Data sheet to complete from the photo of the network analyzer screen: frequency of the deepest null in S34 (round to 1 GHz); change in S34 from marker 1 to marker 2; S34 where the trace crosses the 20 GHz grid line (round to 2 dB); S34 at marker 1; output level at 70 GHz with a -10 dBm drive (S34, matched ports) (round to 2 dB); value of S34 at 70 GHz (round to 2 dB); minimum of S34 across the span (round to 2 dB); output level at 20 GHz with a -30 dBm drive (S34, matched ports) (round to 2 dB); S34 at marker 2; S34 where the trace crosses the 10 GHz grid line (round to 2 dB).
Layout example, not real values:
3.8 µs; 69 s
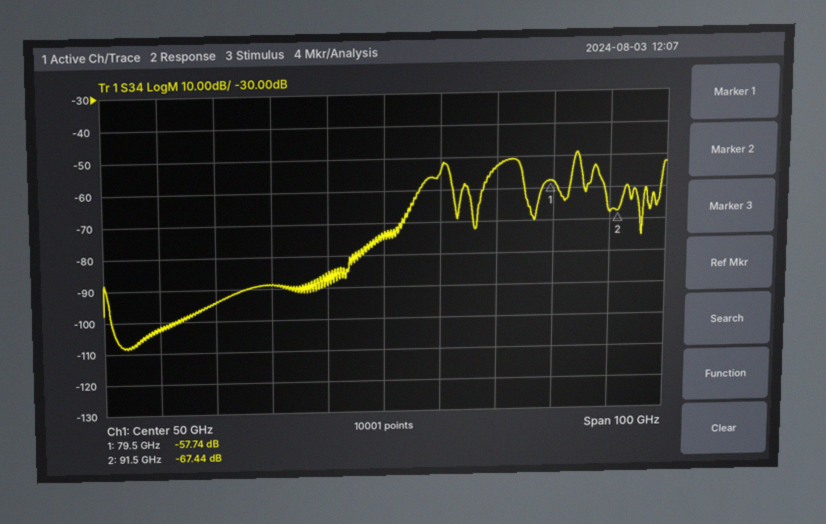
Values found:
4 GHz; -9.70 dB; -94 dB; -57.74 dB; -62 dBm; -52 dB; -108 dB; -124 dBm; -67.44 dB; -102 dB
